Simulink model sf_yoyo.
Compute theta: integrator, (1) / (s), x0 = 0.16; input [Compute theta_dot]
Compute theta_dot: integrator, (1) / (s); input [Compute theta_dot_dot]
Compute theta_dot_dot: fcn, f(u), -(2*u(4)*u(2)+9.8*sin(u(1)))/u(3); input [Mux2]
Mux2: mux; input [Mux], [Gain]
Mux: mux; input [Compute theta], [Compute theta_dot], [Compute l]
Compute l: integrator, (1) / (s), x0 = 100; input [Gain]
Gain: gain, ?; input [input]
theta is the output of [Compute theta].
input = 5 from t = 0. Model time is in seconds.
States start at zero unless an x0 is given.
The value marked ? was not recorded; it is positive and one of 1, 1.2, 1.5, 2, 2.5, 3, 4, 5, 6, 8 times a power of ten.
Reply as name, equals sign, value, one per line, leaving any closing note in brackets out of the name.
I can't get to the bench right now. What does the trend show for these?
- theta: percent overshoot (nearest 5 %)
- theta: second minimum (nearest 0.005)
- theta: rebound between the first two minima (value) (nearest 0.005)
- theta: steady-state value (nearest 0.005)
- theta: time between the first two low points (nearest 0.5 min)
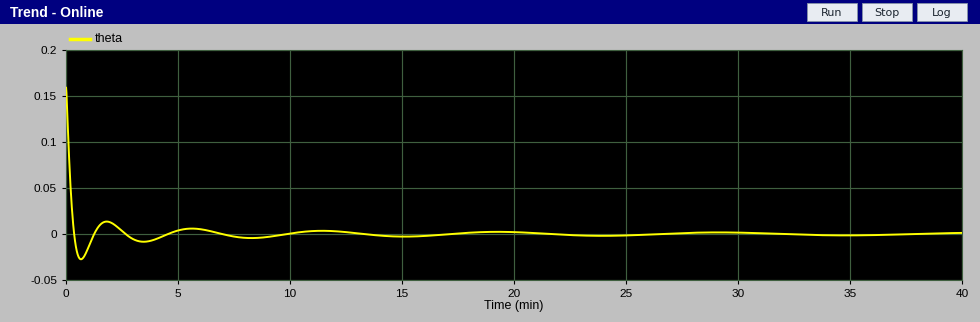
theta: percent overshoot = 15 %
theta: second minimum = -0.010
theta: rebound between the first two minima (value) = 0.015
theta: steady-state value = 0.000
theta: time between the first two low points = 3.0 min
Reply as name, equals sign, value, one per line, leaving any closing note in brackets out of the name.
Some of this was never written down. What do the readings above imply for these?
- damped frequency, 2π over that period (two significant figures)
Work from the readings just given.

damped frequency, 2π over that period = 2.1 rad/min
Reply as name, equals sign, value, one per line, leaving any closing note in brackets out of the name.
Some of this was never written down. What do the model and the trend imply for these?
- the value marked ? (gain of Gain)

the value marked ? = 12
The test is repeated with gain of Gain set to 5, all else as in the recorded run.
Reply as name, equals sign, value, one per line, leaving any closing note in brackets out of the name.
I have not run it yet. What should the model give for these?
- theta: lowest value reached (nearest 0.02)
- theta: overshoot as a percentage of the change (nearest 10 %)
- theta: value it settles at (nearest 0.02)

theta: lowest value reached = -0.04
theta: overshoot as a percentage of the change = 30 %
theta: value it settles at = 0.00
